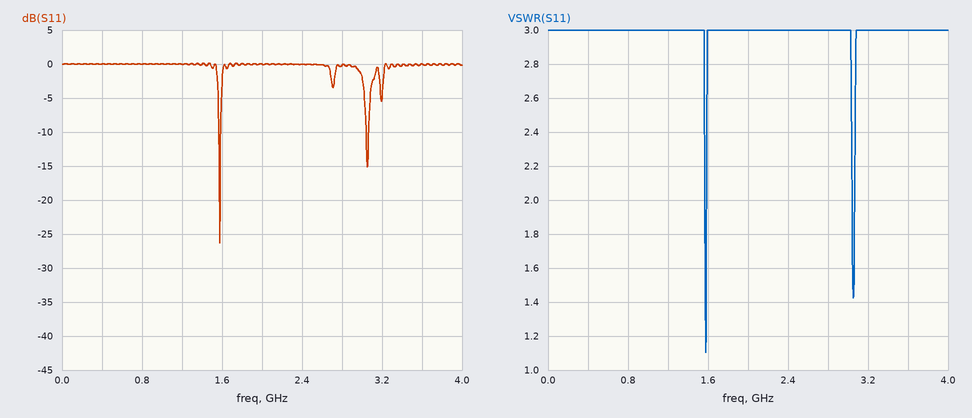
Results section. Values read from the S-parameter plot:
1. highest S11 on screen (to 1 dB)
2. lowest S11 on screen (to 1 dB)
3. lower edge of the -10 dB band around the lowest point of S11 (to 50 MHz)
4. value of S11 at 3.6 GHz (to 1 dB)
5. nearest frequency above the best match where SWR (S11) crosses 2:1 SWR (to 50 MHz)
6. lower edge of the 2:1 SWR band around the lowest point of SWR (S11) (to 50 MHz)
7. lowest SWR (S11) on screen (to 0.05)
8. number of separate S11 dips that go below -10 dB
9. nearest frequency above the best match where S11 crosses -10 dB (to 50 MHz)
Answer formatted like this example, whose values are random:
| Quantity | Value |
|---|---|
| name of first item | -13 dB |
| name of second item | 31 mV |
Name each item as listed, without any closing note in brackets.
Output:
| Quantity | Value |
|---|---|
| highest S11 on screen | 0 dB |
| lowest S11 on screen | -26 dB |
| lower edge of the -10 dB band around the lowest point of S11 | 1.55 GHz |
| value of S11 at 3.6 GHz | 0 dB |
| nearest frequency above the best match where SWR (S11) crosses 2:1 SWR | 1.60 GHz |
| lower edge of the 2:1 SWR band around the lowest point of SWR (S11) | 1.55 GHz |
| lowest SWR (S11) on screen | 1.10 |
| number of separate S11 dips that go below -10 dB | 2 |
| nearest frequency above the best match where S11 crosses -10 dB | 1.60 GHz |
